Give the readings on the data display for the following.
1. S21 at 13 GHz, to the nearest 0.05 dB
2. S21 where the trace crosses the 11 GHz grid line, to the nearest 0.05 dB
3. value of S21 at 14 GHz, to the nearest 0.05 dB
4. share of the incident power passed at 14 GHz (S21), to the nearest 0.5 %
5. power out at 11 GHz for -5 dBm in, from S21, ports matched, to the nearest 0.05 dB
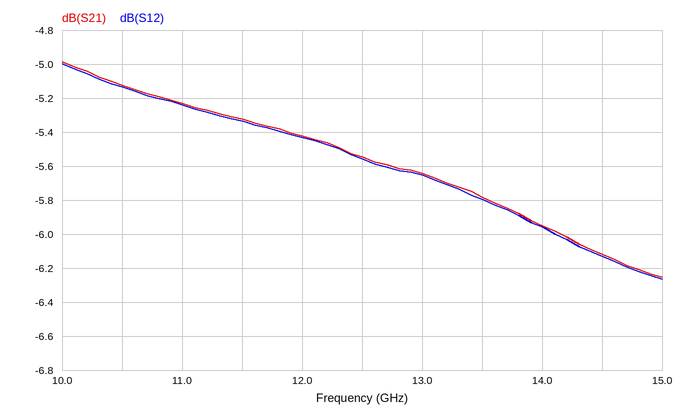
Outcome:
-5.65 dB
-5.25 dB
-5.95 dB
25.5 %
-10.25 dBm
